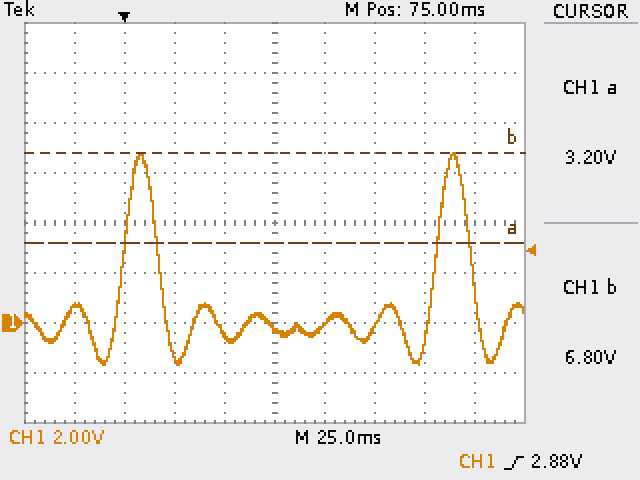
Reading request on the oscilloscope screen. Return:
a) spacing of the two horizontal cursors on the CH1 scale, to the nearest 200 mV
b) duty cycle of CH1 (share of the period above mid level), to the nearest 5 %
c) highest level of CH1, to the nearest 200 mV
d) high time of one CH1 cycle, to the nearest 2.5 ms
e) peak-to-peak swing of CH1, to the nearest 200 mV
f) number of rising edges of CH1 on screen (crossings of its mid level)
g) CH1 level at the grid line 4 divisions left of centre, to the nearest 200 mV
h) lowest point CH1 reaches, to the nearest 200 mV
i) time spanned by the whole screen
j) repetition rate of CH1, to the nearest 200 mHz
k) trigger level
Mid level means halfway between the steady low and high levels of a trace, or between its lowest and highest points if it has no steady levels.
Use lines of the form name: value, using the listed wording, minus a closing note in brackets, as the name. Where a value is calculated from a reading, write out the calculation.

spacing of the two horizontal cursors on the CH1 scale, to the nearest 200 mV: 3.6 V
duty cycle of CH1 (share of the period above mid level), to the nearest 5 %: 10 %
highest level of CH1, to the nearest 200 mV: 6.8 V
high time of one CH1 cycle, to the nearest 2.5 ms: 17.5 ms
peak-to-peak swing of CH1, to the nearest 200 mV: 6.8 V − (-1.6 V) = 8.4 V
number of rising edges of CH1 on screen: 2
CH1 level at the grid line 4 divisions left of centre, to the nearest 200 mV: 600 mV
lowest point CH1 reaches, to the nearest 200 mV: -1.6 V
time spanned by the whole screen: 250 ms
repetition rate of CH1, to the nearest 200 mHz: 6.4 Hz
trigger level: 2.88 V
